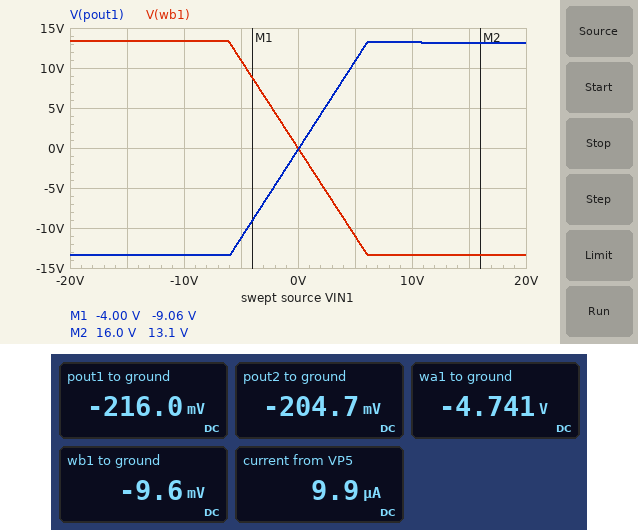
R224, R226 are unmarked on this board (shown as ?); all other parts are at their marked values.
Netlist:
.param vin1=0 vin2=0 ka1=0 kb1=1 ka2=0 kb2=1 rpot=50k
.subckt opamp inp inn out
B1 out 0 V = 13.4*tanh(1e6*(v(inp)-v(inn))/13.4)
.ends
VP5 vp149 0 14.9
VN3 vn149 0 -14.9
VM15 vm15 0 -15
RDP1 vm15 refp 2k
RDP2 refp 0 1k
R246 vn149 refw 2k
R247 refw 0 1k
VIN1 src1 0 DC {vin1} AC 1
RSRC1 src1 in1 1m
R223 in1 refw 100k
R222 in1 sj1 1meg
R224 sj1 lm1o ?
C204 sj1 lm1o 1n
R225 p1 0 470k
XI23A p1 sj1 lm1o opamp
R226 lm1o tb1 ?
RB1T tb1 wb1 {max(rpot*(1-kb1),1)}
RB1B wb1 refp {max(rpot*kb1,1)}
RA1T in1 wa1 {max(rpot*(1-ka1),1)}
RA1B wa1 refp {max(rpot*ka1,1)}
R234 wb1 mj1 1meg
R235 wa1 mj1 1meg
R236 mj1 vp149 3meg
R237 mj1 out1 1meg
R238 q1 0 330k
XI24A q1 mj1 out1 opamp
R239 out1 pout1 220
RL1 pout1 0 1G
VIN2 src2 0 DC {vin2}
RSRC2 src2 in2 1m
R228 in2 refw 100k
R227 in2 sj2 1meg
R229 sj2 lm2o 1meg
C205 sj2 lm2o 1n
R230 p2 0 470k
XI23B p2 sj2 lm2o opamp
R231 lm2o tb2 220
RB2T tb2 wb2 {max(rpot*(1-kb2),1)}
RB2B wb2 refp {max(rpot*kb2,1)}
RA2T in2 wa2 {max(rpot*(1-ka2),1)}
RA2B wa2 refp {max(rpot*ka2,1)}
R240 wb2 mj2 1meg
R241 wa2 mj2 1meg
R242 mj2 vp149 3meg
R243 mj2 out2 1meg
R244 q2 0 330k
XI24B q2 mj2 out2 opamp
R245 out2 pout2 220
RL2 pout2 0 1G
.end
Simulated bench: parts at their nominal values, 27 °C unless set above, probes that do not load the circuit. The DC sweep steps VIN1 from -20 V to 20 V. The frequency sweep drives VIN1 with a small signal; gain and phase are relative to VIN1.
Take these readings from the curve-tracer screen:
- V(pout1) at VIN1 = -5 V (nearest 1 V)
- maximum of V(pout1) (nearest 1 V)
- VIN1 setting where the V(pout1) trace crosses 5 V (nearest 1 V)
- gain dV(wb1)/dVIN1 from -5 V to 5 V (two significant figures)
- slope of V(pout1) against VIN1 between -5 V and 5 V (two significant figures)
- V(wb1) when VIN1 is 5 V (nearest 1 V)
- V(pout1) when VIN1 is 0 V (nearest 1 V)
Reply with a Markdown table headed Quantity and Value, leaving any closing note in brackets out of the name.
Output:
| Quantity | Value |
|---|---|
| V(pout1) at VIN1 = -5 V | -11 V |
| maximum of V(pout1) | 13 V |
| VIN1 setting where the V(pout1) trace crosses 5 V | 2 V |
| gain dV(wb1)/dVIN1 from -5 V to 5 V | -2.2 V/V |
| slope of V(pout1) against VIN1 between -5 V and 5 V | 2.2 V/V |
| V(wb1) when VIN1 is 5 V | -11 V |
| V(pout1) when VIN1 is 0 V | 0 V |
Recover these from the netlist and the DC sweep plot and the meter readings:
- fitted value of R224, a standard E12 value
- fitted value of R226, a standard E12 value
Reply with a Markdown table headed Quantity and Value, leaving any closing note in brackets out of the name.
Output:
| Quantity | Value |
|---|---|
| fitted value of R224, a standard E12 value | 2.2 MΩ |
| fitted value of R226, a standard E12 value | 100 Ω |
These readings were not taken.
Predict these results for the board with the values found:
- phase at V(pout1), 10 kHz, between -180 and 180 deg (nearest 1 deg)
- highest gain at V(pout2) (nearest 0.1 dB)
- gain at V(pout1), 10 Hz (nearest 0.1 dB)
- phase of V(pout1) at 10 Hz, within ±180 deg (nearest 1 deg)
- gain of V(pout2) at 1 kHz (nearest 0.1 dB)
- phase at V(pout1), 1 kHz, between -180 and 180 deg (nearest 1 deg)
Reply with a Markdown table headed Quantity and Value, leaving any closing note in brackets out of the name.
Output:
| Quantity | Value |
|---|---|
| phase at V(pout1), 10 kHz, between -180 and 180 deg | -128 deg |
| highest gain at V(pout2) | -36.4 dB |
| gain at V(pout1), 10 Hz | 6.8 dB |
| phase of V(pout1) at 10 Hz, within ±180 deg | -8 deg |
| gain of V(pout2) at 1 kHz | -37.9 dB |
| phase at V(pout1), 1 kHz, between -180 and 180 deg | -90 deg |
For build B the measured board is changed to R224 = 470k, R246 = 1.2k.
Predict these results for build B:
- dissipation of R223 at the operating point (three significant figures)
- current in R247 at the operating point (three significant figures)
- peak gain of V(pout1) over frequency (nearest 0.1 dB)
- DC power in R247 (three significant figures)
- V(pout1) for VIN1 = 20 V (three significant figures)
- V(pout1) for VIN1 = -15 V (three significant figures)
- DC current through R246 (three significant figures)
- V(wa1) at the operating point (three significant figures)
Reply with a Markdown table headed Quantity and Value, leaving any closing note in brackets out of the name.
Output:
| Quantity | Value |
|---|---|
| dissipation of R223 at the operating point | 449 µW |
| current in R247 at the operating point | 6.70 mA |
| peak gain of V(pout1) over frequency | -6.7 dB |
| DC power in R247 | 44.9 mW |
| V(pout1) for VIN1 = 20 V | 9.03 V |
| V(pout1) for VIN1 = -15 V | -7.15 V |
| DC current through R246 | 6.83 mA |
| V(wa1) at the operating point | -4.74 V |
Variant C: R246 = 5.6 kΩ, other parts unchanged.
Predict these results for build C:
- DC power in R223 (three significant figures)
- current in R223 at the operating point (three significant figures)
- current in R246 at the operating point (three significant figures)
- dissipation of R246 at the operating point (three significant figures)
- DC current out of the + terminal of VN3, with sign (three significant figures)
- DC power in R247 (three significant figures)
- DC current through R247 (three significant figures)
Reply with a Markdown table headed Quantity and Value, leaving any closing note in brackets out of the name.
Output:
| Quantity | Value |
|---|---|
| DC power in R223 | 49.3 µW |
| current in R223 at the operating point | 22.2 µA |
| current in R246 at the operating point | 2.26 mA |
| dissipation of R246 at the operating point | 28.7 mW |
| DC current out of the + terminal of VN3, with sign | -2.26 mA |
| DC power in R247 | 4.93 mW |
| DC current through R247 | 2.22 mA |
